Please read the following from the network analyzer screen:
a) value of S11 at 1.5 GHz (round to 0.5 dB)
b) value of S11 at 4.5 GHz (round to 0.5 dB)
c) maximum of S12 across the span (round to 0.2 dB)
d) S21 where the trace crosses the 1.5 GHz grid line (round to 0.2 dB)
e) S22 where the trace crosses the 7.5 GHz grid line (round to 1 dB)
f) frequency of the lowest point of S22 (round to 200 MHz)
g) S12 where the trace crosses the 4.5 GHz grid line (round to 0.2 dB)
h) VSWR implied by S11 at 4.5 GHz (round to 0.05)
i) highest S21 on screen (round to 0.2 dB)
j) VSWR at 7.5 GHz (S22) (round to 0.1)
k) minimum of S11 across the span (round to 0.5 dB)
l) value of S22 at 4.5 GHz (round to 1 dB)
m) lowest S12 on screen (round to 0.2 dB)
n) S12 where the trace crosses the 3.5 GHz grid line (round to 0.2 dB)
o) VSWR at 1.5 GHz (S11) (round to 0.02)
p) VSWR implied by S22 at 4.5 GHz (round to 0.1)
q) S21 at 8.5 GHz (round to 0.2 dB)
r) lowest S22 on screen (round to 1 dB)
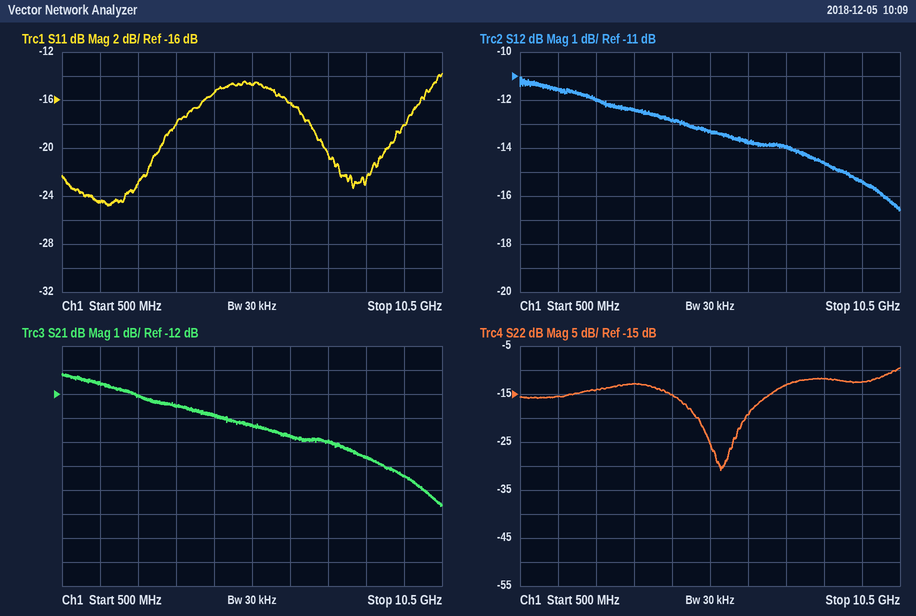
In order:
-24.5 dB
-15.5 dB
-11.0 dB
-11.6 dB
-13 dB
5.8 GHz
-12.8 dB
1.40
-11.2 dB
1.6
-25.0 dB
-15 dB
-16.6 dB
-12.4 dB
1.12
1.4
-14.6 dB
-31 dB
